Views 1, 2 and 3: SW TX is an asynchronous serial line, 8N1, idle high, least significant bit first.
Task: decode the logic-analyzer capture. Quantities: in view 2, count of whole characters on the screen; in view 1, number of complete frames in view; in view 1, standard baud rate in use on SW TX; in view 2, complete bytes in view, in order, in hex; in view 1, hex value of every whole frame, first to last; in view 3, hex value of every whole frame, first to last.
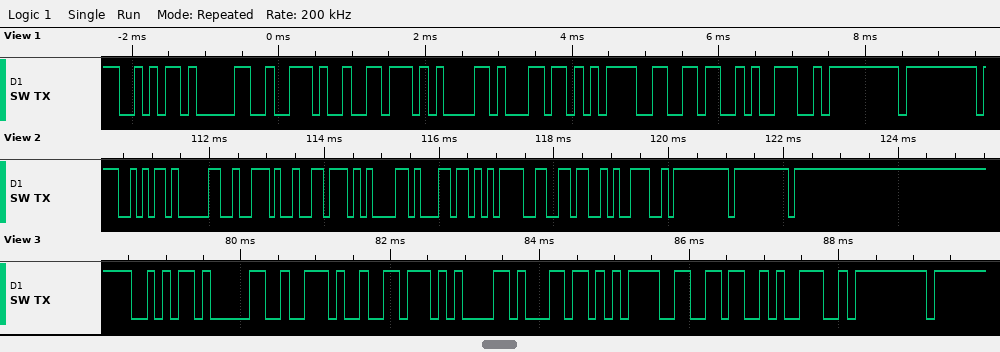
12
11
9600 baud
0x6A 0x30 0x2E 0x76 0x61 0x6C 0x3D 0x36 0x39 0xFF 0xFF 0xFF
6A 30 2E 76 61 6C 3D 36 39 FF FF
6A 30 2E 76 61 6C 3D 36 39 FF
